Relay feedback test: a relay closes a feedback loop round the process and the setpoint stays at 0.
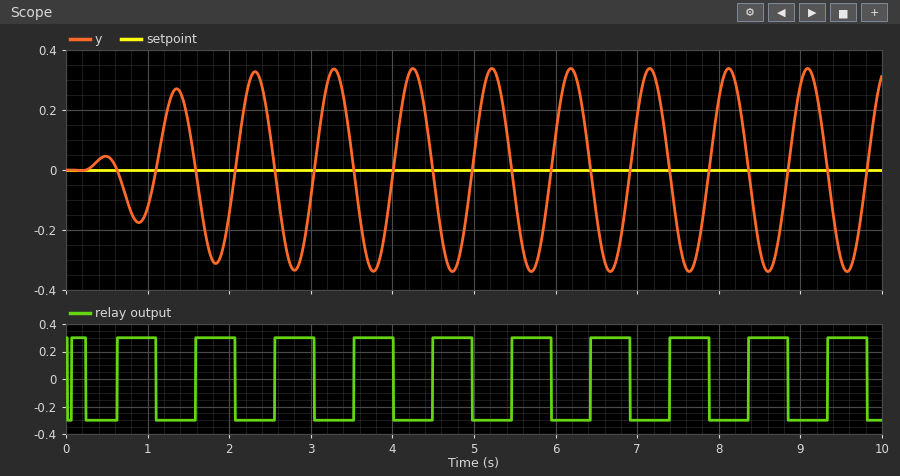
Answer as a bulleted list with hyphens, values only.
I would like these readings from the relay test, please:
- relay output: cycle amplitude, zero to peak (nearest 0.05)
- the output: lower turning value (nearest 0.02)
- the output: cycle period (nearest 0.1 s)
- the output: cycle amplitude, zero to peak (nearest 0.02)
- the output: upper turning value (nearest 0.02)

- 0.30
- -0.34
- 1.0 s
- 0.34
- 0.34
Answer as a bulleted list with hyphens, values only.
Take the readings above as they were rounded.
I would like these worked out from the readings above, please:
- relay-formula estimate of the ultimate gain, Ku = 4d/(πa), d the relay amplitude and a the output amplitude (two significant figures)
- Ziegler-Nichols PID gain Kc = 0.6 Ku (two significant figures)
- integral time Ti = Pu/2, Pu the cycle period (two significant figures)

- 1.1
- 0.66
- 0.50 s
